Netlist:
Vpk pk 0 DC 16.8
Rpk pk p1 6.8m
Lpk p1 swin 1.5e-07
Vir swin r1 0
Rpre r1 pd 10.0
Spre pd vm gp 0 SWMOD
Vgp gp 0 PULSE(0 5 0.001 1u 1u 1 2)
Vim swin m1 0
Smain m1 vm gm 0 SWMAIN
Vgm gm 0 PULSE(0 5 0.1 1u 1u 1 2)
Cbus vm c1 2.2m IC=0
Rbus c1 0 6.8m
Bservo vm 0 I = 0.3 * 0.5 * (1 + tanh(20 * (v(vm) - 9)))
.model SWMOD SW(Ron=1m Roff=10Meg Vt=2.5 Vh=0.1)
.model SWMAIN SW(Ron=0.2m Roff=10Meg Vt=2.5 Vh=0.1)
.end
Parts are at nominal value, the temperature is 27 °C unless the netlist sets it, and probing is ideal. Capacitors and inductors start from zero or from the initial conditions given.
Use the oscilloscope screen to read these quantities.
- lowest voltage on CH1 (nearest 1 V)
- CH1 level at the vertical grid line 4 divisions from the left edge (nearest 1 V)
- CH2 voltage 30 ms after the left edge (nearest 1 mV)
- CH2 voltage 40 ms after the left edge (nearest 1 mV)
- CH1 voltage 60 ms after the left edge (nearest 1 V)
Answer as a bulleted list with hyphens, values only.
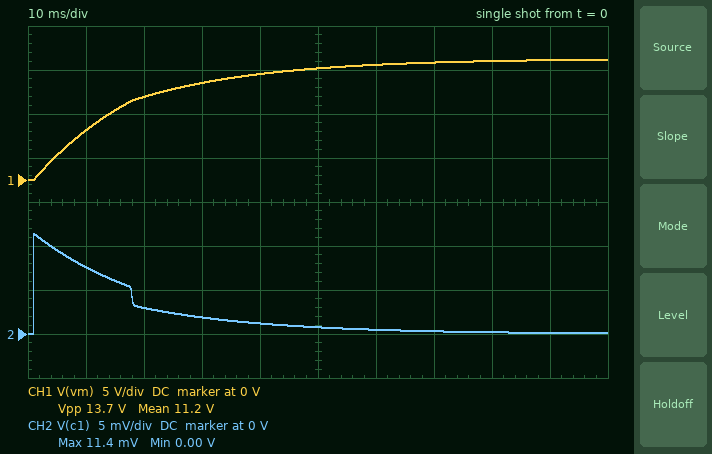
- 0 V
- 12 V
- 2 mV
- 1 mV
- 13 V
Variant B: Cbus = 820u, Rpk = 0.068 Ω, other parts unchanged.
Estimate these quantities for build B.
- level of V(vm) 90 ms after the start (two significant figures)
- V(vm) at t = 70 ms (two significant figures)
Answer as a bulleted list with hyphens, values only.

- 14 V
- 14 V
